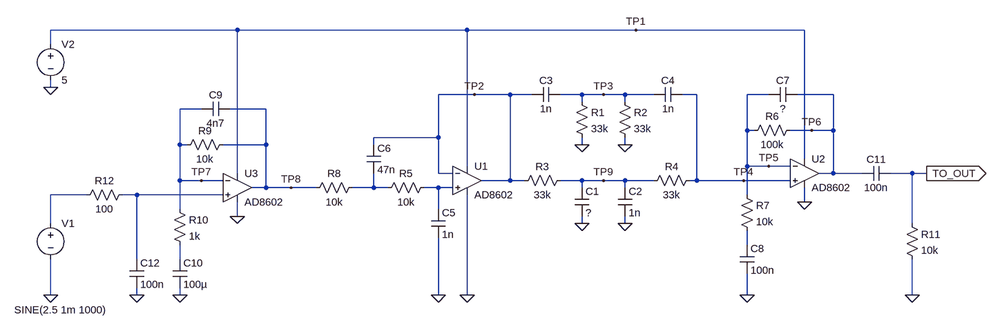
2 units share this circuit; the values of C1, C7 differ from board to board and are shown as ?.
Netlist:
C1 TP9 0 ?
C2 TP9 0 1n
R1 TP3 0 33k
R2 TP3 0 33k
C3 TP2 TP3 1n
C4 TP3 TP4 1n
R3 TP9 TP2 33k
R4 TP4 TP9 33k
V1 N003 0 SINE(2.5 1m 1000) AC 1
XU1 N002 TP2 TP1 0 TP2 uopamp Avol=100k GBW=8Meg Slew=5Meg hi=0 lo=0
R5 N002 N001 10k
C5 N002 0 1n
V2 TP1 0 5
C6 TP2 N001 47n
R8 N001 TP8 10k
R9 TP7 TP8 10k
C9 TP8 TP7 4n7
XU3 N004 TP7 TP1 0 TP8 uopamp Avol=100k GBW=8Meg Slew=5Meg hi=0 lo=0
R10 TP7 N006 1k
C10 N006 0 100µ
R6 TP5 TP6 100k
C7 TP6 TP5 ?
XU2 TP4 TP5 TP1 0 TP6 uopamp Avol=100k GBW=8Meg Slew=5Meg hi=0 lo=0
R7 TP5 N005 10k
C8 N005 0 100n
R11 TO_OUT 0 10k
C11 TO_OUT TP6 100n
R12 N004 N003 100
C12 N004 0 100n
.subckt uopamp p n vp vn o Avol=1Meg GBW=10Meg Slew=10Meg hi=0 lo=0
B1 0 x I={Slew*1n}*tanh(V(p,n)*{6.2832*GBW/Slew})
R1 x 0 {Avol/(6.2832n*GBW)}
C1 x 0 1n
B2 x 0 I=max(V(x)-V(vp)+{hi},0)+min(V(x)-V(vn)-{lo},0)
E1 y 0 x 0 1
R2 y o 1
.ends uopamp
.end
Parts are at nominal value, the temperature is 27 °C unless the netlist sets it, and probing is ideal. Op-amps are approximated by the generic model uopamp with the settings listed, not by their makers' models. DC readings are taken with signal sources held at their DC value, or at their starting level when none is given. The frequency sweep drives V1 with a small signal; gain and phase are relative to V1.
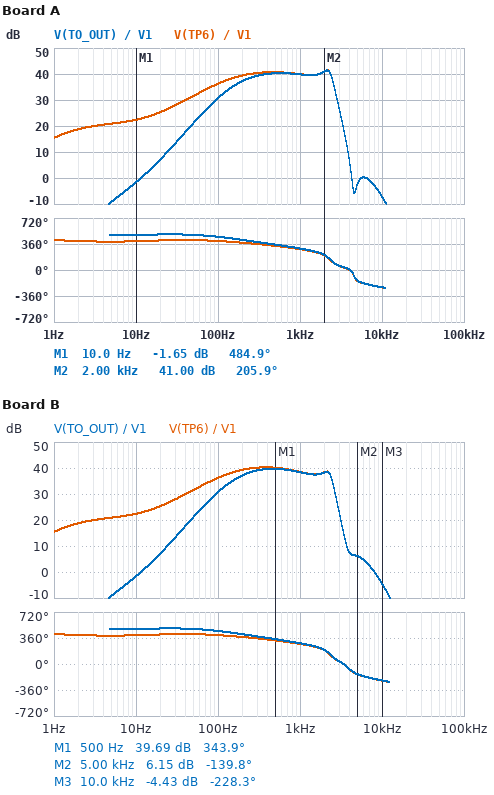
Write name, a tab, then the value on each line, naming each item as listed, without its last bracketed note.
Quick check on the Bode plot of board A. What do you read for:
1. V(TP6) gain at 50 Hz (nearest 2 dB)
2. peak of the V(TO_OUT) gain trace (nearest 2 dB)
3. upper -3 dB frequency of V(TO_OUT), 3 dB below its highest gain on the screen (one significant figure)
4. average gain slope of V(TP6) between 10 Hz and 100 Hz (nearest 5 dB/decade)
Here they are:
V(TP6) gain at 50 Hz	32 dB
peak of the V(TO_OUT) gain trace	42 dB
upper -3 dB frequency of V(TO_OUT), 3 dB below its highest gain on the screen	2 kHz
average gain slope of V(TP6) between 10 Hz and 100 Hz	15 dB/decade
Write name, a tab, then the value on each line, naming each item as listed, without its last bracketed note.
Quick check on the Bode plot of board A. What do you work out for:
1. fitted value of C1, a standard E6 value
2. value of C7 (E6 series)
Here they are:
fitted value of C1, a standard E6 value	1.5 nF
value of C7	220 pF
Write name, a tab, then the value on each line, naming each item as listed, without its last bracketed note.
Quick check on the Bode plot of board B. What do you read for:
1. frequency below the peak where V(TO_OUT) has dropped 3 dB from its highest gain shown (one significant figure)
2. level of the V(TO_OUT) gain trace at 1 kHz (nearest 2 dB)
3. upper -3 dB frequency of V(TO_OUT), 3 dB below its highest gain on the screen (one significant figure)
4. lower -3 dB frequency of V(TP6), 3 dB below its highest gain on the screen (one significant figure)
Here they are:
frequency below the peak where V(TO_OUT) has dropped 3 dB from its highest gain shown	200 Hz
level of the V(TO_OUT) gain trace at 1 kHz	38 dB
upper -3 dB frequency of V(TO_OUT), 3 dB below its highest gain on the screen	2 kHz
lower -3 dB frequency of V(TP6), 3 dB below its highest gain on the screen	100 Hz
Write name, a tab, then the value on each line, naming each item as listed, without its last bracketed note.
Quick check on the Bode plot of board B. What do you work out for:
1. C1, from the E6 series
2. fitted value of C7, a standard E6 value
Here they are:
C1, from the E6 series	3.3 nF
fitted value of C7, a standard E6 value	150 pF
